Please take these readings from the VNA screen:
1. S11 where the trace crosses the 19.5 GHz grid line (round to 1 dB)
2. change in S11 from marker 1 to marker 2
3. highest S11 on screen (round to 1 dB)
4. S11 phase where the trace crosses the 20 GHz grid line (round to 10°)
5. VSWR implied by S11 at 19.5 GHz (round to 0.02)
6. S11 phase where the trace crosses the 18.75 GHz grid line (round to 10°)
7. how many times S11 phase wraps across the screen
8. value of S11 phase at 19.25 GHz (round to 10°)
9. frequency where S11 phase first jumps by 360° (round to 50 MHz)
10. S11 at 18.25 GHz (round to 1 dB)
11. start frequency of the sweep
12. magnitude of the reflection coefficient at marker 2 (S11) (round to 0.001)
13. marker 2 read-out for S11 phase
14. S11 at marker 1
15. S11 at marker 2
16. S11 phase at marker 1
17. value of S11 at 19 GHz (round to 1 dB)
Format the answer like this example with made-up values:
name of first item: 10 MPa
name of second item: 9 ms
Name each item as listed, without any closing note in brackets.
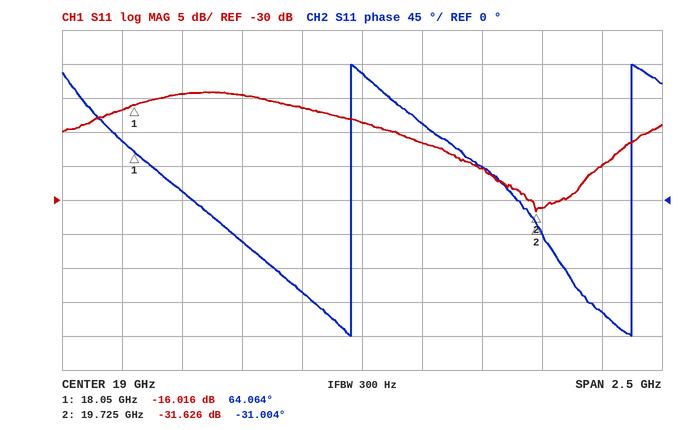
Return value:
S11 where the trace crosses the 19.5 GHz grid line: -25 dB
change in S11 from marker 1 to marker 2: -15.610 dB
highest S11 on screen: -14 dB
S11 phase where the trace crosses the 20 GHz grid line: -150°
VSWR implied by S11 at 19.5 GHz: 1.12
S11 phase where the trace crosses the 18.75 GHz grid line: -120°
how many times S11 phase wraps across the screen: 2
value of S11 phase at 19.25 GHz: 100°
frequency where S11 phase first jumps by 360°: 18.95 GHz
S11 at 18.25 GHz: -14 dB
start frequency of the sweep: 17.75 GHz
magnitude of the reflection coefficient at marker 2 (S11): 0.026
marker 2 read-out for S11 phase: -31.004°
S11 at marker 1: -16.016 dB
S11 at marker 2: -31.626 dB
S11 phase at marker 1: 64.064°
value of S11 at 19 GHz: -19 dB
